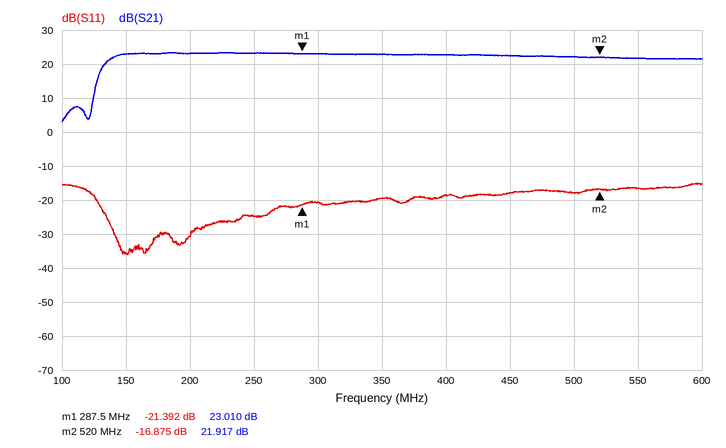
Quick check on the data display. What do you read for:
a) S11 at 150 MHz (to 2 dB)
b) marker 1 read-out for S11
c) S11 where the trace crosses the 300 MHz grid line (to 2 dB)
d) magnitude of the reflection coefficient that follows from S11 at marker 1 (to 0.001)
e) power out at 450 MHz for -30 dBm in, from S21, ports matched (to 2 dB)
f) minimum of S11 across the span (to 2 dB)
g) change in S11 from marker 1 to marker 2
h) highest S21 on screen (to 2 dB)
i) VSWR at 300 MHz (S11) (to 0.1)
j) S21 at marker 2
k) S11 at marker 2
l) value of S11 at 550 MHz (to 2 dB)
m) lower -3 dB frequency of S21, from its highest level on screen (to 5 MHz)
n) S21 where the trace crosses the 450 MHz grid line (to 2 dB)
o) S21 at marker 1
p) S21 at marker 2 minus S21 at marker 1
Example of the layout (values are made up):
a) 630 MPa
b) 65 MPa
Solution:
a) -36 dB
b) -21.392 dB
c) -20 dB
d) 0.085
e) -8 dBm
f) -36 dB
g) 4.517 dB
h) 24 dB
i) 1.2
j) 21.917 dB
k) -16.875 dB
l) -16 dB
m) 135 MHz
n) 22 dB
o) 23.010 dB
p) -1.093 dB
